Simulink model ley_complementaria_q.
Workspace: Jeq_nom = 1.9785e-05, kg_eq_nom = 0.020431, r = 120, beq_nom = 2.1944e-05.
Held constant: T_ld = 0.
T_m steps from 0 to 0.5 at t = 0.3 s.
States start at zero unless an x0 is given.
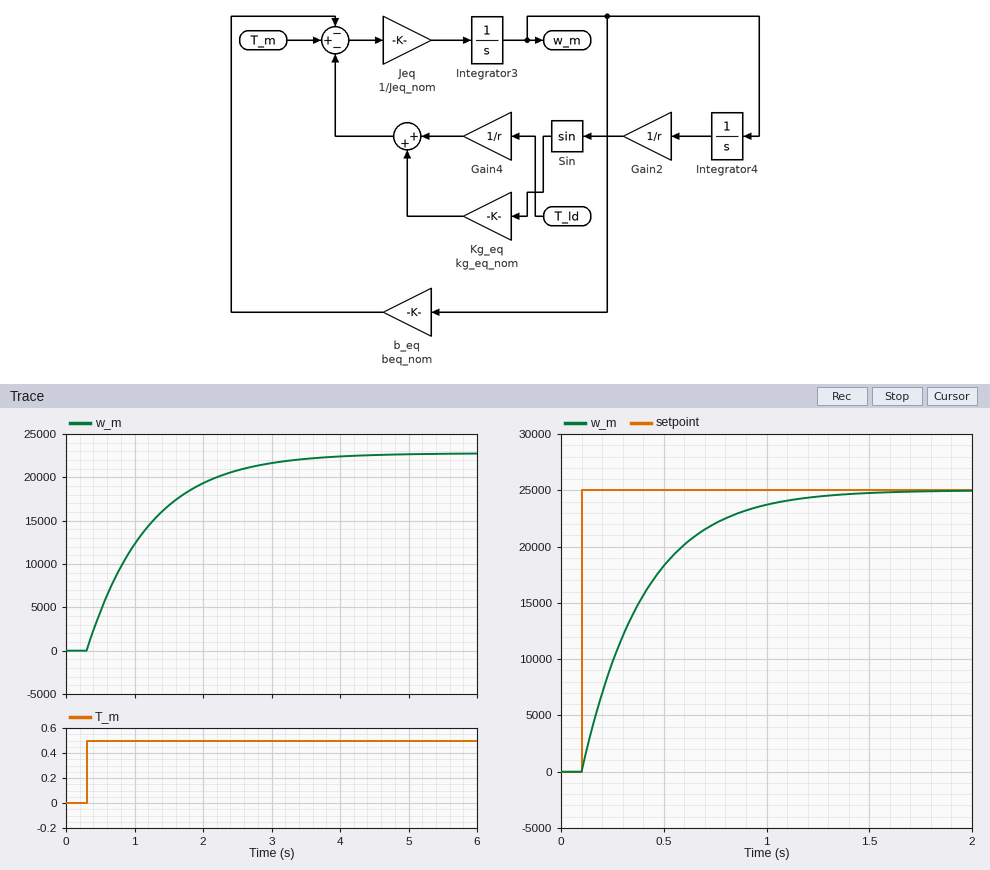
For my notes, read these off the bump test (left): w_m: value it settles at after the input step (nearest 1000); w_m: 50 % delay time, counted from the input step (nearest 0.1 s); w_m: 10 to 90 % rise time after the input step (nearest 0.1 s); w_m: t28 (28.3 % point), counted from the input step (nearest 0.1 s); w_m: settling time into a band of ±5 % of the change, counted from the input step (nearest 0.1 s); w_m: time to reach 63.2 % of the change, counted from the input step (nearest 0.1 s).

23000
0.6 s
2.0 s
0.3 s
2.7 s
0.9 s
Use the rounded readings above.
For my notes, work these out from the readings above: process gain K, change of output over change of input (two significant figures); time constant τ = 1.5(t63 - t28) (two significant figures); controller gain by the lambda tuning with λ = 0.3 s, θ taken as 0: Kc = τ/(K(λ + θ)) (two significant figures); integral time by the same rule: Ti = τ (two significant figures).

46000
0.90 s
0.000065
0.90 s
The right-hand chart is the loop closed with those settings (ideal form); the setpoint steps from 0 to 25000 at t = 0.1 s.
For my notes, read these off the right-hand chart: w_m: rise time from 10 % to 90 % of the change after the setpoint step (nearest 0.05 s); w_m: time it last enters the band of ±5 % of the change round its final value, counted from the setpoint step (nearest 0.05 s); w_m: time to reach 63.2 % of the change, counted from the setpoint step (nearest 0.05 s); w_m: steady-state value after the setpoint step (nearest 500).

0.65 s
0.90 s
0.30 s
25000
